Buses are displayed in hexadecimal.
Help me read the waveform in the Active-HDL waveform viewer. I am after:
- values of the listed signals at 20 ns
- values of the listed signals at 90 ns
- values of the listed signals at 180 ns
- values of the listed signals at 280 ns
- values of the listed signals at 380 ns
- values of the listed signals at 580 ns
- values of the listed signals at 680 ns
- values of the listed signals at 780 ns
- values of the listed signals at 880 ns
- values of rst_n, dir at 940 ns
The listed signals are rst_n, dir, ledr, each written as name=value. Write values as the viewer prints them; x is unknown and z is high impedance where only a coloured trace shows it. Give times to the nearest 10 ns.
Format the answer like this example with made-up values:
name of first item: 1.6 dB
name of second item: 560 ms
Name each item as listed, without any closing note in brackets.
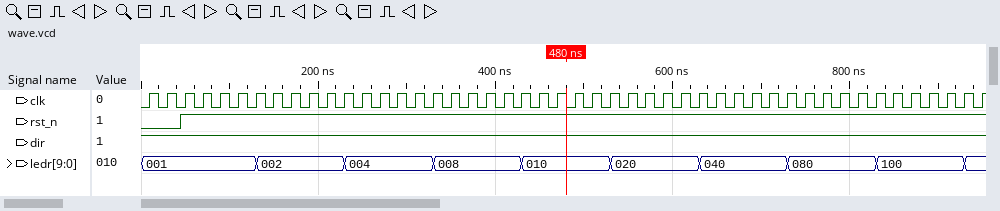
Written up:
values of the listed signals at 20 ns: rst_n=0, dir=1, ledr=001
values of the listed signals at 90 ns: rst_n=1, dir=1, ledr=001
values of the listed signals at 180 ns: rst_n=1, dir=1, ledr=002
values of the listed signals at 280 ns: rst_n=1, dir=1, ledr=004
values of the listed signals at 380 ns: rst_n=1, dir=1, ledr=008
values of the listed signals at 580 ns: rst_n=1, dir=1, ledr=020
values of the listed signals at 680 ns: rst_n=1, dir=1, ledr=040
values of the listed signals at 780 ns: rst_n=1, dir=1, ledr=080
values of the listed signals at 880 ns: rst_n=1, dir=1, ledr=100
values of rst_n, dir at 940 ns: rst_n=1, dir=1
